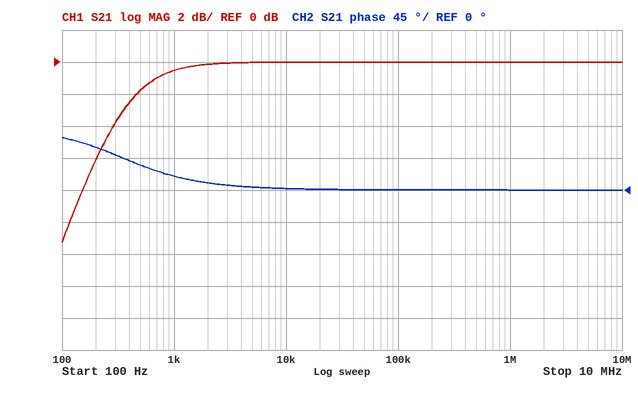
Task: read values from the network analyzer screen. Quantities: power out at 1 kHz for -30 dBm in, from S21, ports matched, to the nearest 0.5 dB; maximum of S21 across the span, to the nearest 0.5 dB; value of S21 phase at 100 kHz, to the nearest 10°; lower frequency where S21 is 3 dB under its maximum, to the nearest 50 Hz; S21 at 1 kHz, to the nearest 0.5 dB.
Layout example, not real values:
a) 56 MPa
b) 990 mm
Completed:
a) -30.5 dBm
b) 0.0 dB
c) 0°
d) 350 Hz
e) -0.5 dB
